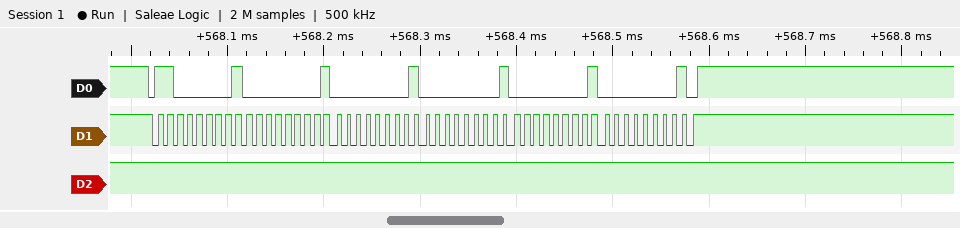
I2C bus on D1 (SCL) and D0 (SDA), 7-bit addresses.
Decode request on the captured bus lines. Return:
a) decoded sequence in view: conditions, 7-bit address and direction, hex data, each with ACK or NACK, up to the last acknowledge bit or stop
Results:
start, address 60 write NACK, 00 NACK, 00 NACK, 00 NACK, 00 NACK, 00 NACK, stop
